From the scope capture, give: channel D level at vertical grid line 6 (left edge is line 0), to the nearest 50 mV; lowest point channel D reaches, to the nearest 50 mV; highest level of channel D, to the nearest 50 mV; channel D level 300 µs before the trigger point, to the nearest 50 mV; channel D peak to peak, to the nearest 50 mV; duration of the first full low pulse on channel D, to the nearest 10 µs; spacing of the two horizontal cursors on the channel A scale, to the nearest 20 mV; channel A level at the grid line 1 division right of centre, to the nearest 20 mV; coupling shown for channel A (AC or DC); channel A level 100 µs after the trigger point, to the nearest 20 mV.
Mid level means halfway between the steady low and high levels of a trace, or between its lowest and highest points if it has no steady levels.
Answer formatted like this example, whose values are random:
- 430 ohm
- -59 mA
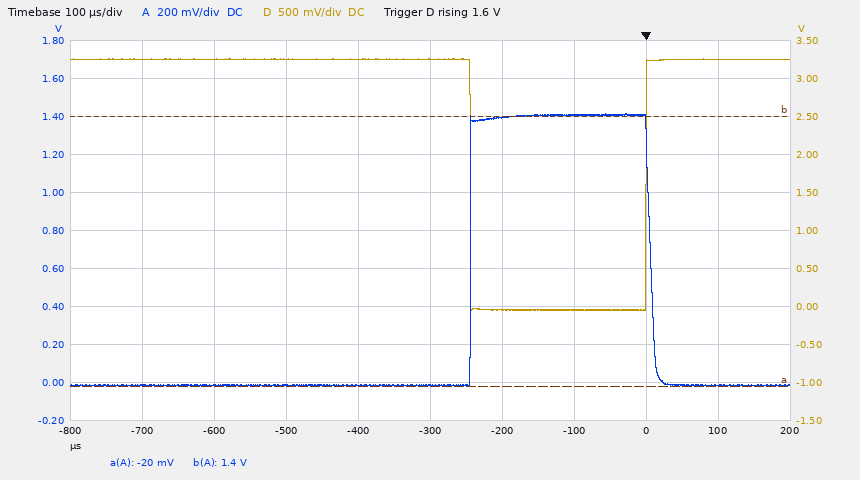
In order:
- -50 mV
- -50 mV
- 3.25 V
- 3.25 V
- 3.30 V
- 240 µs
- 1.42 V
- 1.40 V
- DC
- -20 mV
